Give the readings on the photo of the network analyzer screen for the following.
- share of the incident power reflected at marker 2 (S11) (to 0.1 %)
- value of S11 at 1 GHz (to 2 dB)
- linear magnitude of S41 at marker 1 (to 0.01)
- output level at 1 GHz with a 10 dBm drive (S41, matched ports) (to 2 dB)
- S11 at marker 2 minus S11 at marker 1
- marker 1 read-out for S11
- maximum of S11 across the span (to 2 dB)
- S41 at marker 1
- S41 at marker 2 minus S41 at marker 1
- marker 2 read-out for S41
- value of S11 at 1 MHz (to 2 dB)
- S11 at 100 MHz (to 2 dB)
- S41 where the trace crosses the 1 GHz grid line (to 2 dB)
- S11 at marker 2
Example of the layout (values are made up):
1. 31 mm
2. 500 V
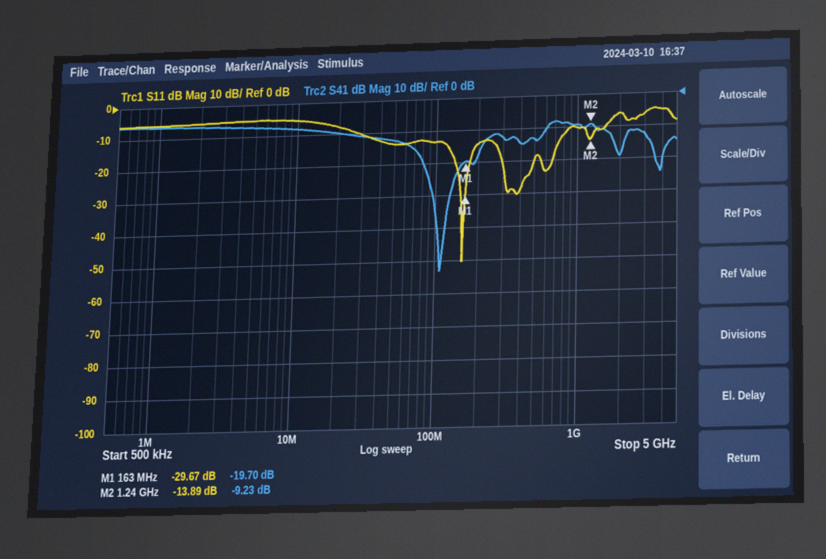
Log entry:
1. 4.1 %
2. -10 dB
3. 0.10
4. 0 dBm
5. 15.78 dB
6. -29.67 dB
7. -4 dB
8. -19.70 dB
9. 10.47 dB
10. -9.23 dB
11. -6 dB
12. -14 dB
13. -10 dB
14. -13.89 dB
